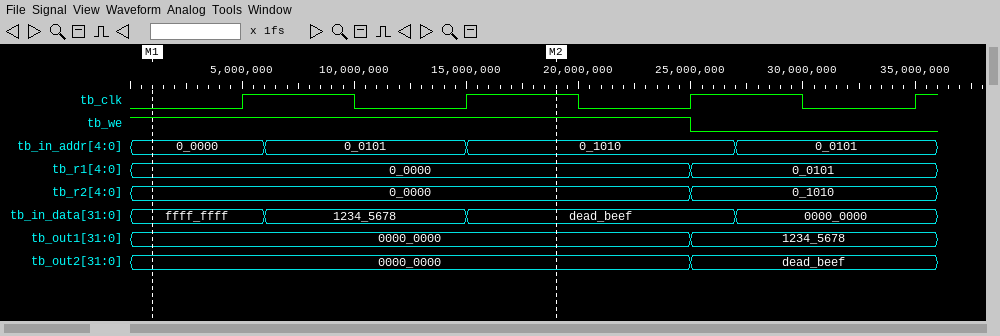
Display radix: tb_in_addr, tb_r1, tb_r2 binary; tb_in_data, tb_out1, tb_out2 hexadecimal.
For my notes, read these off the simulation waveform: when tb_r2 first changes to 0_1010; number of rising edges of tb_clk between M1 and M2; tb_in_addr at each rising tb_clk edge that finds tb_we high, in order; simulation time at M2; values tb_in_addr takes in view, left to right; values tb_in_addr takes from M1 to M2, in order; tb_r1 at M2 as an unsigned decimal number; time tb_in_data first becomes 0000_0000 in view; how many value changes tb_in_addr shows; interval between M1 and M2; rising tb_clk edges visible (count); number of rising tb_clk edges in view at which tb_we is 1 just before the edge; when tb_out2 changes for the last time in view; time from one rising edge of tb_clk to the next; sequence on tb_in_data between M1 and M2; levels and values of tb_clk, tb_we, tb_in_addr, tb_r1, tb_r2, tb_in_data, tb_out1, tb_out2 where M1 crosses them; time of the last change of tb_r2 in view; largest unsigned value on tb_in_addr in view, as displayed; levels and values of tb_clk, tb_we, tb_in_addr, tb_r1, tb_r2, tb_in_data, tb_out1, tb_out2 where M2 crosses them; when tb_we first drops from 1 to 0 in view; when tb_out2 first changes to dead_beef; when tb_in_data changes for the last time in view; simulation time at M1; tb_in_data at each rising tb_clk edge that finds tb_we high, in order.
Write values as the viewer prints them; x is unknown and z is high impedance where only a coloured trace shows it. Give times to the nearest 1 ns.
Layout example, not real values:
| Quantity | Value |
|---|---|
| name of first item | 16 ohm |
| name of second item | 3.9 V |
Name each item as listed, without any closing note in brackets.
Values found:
| Quantity | Value |
|---|---|
| when tb_r2 first changes to 0_1010 | 25 ns |
| number of rising edges of tb_clk between M1 and M2 | 2 |
| tb_in_addr at each rising tb_clk edge that finds tb_we high, in order | 0_0000, 0_0101, 0_1010 |
| simulation time at M2 | 19 ns |
| values tb_in_addr takes in view, left to right | 0_0000, 0_0101, 0_1010, 0_0101 |
| values tb_in_addr takes from M1 to M2, in order | 0_0000, 0_0101, 0_1010 |
| tb_r1 at M2 as an unsigned decimal number | 0 |
| time tb_in_data first becomes 0000_0000 in view | 27 ns |
| how many value changes tb_in_addr shows | 3 |
| interval between M1 and M2 | 18 ns |
| rising tb_clk edges visible | 4 |
| number of rising tb_clk edges in view at which tb_we is 1 just before the edge | 3 |
| when tb_out2 changes for the last time in view | 25 ns |
| time from one rising edge of tb_clk to the next | 10 ns |
| sequence on tb_in_data between M1 and M2 | ffff_ffff, 1234_5678, dead_beef |
| levels and values of tb_clk, tb_we, tb_in_addr, tb_r1, tb_r2, tb_in_data, tb_out1, tb_out2 where M1 crosses them | tb_clk=0, tb_we=1, tb_in_addr=0_0000, tb_r1=0_0000, tb_r2=0_0000, tb_in_data=ffff_ffff, tb_out1=0000_0000, tb_out2=0000_0000 |
| time of the last change of tb_r2 in view | 25 ns |
| largest unsigned value on tb_in_addr in view, as displayed | 0_1010 |
| levels and values of tb_clk, tb_we, tb_in_addr, tb_r1, tb_r2, tb_in_data, tb_out1, tb_out2 where M2 crosses them | tb_clk=1, tb_we=1, tb_in_addr=0_1010, tb_r1=0_0000, tb_r2=0_0000, tb_in_data=dead_beef, tb_out1=0000_0000, tb_out2=0000_0000 |
| when tb_we first drops from 1 to 0 in view | 25 ns |
| when tb_out2 first changes to dead_beef | 25 ns |
| when tb_in_data changes for the last time in view | 27 ns |
| simulation time at M1 | 1 ns |
| tb_in_data at each rising tb_clk edge that finds tb_we high, in order | ffff_ffff, 1234_5678, dead_beef |
